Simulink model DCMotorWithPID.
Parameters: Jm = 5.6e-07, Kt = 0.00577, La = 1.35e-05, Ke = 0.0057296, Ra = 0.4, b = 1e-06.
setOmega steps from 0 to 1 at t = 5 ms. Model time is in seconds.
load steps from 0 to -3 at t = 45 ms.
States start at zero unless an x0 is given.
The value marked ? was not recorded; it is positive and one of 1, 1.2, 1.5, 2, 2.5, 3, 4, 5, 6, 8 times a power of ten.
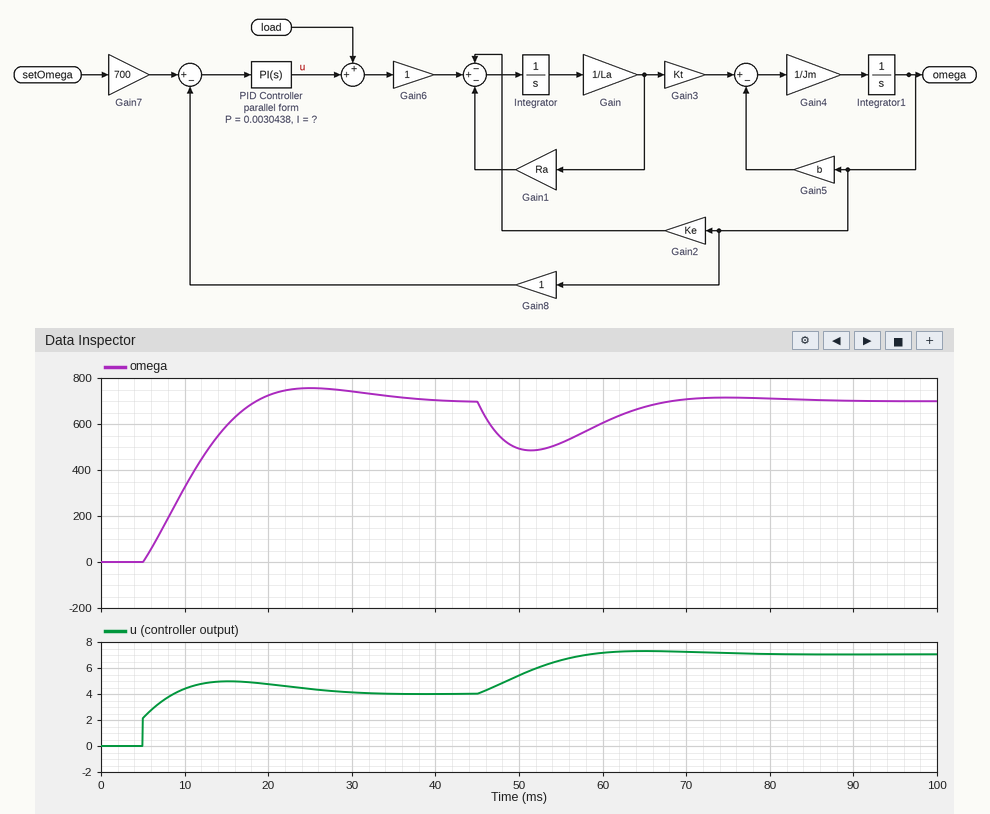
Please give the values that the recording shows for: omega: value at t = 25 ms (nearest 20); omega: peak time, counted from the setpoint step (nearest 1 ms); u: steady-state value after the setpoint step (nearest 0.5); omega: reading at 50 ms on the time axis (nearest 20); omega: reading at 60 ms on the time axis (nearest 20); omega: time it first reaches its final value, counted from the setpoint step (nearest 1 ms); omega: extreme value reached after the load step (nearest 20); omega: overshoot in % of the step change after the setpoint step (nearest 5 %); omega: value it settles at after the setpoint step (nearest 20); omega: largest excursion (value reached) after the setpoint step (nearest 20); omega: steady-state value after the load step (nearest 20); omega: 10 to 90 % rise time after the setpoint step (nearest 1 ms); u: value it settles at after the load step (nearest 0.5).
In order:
760
20 ms
4.0
500
600
14 ms
480
10 %
700
760
700
10 ms
7.0
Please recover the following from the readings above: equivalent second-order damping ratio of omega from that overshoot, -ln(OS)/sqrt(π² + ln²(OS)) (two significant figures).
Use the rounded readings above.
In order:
0.59
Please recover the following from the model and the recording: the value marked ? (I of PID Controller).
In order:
1.2
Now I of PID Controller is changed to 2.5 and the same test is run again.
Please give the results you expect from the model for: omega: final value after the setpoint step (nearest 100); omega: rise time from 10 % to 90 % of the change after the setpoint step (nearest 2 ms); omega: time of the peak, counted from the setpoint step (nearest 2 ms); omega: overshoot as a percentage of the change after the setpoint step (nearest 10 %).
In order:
700
6 ms
12 ms
20 %
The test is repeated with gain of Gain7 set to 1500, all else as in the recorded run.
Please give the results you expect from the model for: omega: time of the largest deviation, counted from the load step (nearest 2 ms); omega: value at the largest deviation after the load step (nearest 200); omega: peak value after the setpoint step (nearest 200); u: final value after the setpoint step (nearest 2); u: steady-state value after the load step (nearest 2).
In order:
6 ms
1200
1600
8
12
